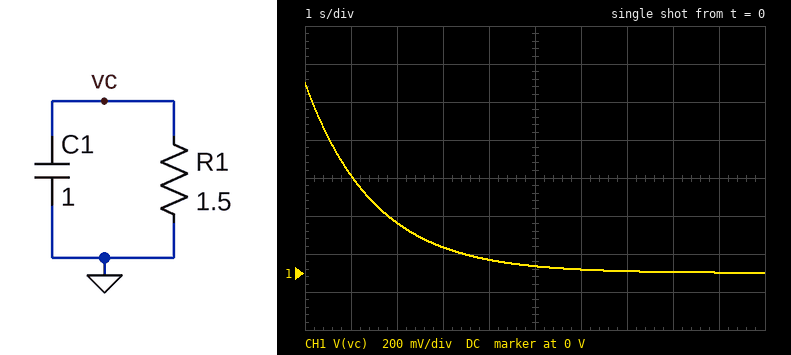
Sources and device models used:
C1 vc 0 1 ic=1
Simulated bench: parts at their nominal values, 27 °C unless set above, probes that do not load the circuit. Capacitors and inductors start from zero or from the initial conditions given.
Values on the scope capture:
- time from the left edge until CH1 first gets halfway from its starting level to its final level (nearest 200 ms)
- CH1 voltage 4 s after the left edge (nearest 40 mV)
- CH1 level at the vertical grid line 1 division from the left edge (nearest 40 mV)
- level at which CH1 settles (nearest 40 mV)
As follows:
1.0 s
80 mV
520 mV
0 V
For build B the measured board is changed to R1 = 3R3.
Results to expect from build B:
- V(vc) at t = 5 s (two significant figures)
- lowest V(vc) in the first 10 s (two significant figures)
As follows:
220 mV
48 mV
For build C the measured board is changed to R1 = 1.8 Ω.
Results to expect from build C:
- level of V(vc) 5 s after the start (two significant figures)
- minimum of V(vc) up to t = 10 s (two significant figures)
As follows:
62 mV
3.9 mV
